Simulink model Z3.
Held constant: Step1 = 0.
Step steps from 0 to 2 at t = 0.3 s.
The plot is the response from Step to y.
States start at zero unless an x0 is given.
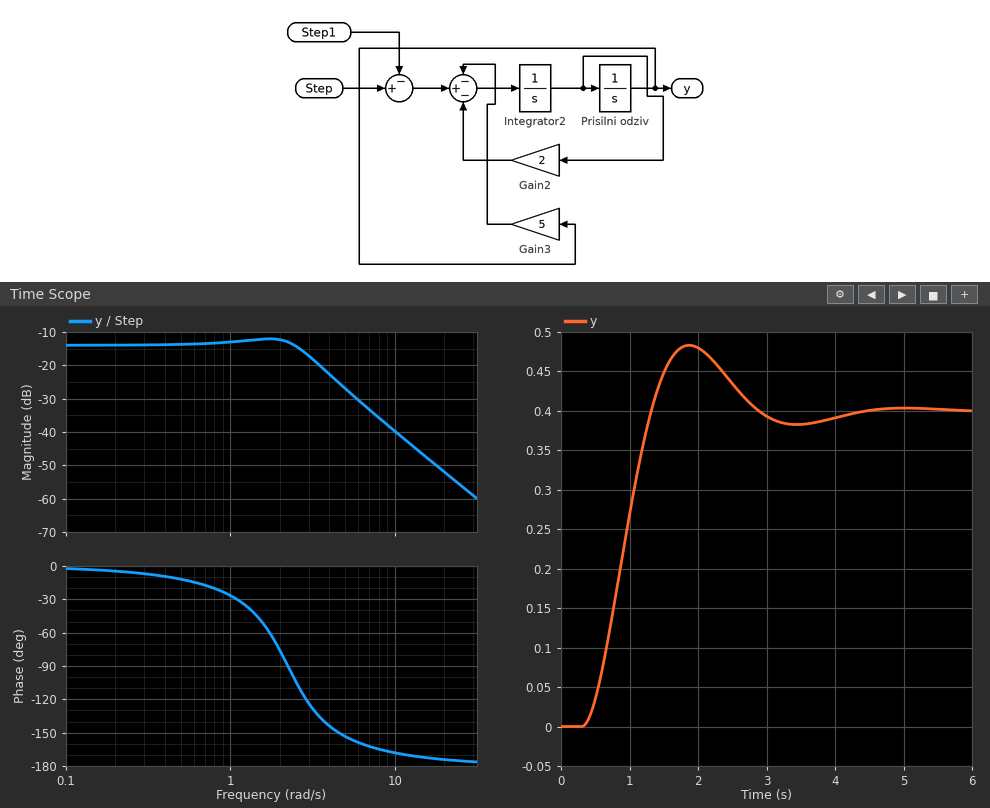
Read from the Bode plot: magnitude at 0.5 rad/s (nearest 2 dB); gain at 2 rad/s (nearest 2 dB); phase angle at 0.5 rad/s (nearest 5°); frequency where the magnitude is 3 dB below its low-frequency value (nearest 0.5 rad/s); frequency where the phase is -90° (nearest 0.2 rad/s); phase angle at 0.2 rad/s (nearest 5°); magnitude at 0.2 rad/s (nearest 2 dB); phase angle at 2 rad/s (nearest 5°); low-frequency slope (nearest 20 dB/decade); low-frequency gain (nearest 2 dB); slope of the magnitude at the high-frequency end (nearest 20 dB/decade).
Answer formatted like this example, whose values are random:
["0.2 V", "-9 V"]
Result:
["-14 dB", "-12 dB", "-10°", "3.0 rad/s", "2.2 rad/s", "-5°", "-14 dB", "-75°", "0 dB/decade", "-14 dB", "-40 dB/decade"]
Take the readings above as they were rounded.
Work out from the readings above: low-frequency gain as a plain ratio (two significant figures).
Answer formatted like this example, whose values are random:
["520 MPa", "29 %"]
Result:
["0.20"]
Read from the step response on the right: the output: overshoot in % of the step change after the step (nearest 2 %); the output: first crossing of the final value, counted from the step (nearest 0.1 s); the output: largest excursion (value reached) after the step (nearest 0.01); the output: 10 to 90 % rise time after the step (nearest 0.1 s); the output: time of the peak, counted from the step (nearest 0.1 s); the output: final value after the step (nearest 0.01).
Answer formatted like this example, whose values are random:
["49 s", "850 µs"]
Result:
["20 %", "1.0 s", "0.48", "0.7 s", "1.6 s", "0.40"]
